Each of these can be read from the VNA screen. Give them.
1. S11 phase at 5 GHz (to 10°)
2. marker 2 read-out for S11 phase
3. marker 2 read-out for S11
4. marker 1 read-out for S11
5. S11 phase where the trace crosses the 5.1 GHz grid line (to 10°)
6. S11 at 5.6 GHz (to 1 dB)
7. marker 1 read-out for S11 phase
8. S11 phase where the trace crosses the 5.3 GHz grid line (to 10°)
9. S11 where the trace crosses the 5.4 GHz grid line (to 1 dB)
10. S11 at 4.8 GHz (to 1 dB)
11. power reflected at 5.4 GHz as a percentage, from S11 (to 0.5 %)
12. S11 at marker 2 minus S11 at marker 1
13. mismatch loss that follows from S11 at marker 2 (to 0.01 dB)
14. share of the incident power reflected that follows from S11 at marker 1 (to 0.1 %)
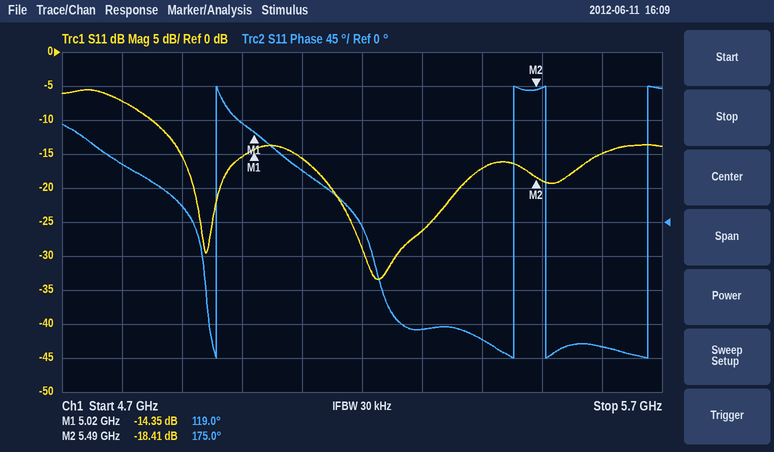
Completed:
130°
175.0°
-18.41 dB
-14.35 dB
70°
-15 dB
119.0°
-140°
-17 dB
-7 dB
2.0 %
-4.06 dB
0.06 dB
3.7 %
